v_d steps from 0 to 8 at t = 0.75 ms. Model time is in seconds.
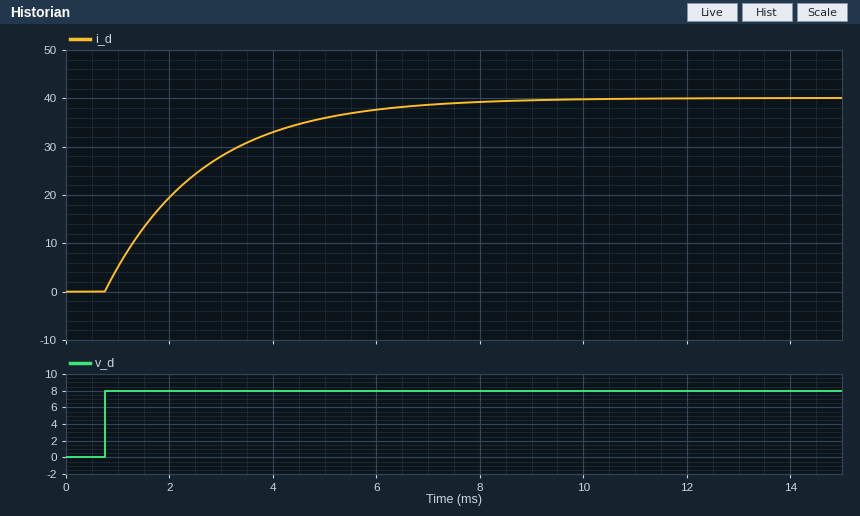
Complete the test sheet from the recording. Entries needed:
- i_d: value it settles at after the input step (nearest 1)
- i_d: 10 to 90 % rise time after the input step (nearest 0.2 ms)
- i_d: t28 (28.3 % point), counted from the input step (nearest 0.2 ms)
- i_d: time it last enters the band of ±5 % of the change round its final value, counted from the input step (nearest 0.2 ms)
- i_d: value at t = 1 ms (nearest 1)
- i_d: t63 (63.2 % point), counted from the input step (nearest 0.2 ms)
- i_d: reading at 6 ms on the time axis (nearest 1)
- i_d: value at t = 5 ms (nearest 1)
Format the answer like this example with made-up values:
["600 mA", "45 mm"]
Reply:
["40", "4.2 ms", "0.6 ms", "5.6 ms", "5", "1.8 ms", "38", "36"]
